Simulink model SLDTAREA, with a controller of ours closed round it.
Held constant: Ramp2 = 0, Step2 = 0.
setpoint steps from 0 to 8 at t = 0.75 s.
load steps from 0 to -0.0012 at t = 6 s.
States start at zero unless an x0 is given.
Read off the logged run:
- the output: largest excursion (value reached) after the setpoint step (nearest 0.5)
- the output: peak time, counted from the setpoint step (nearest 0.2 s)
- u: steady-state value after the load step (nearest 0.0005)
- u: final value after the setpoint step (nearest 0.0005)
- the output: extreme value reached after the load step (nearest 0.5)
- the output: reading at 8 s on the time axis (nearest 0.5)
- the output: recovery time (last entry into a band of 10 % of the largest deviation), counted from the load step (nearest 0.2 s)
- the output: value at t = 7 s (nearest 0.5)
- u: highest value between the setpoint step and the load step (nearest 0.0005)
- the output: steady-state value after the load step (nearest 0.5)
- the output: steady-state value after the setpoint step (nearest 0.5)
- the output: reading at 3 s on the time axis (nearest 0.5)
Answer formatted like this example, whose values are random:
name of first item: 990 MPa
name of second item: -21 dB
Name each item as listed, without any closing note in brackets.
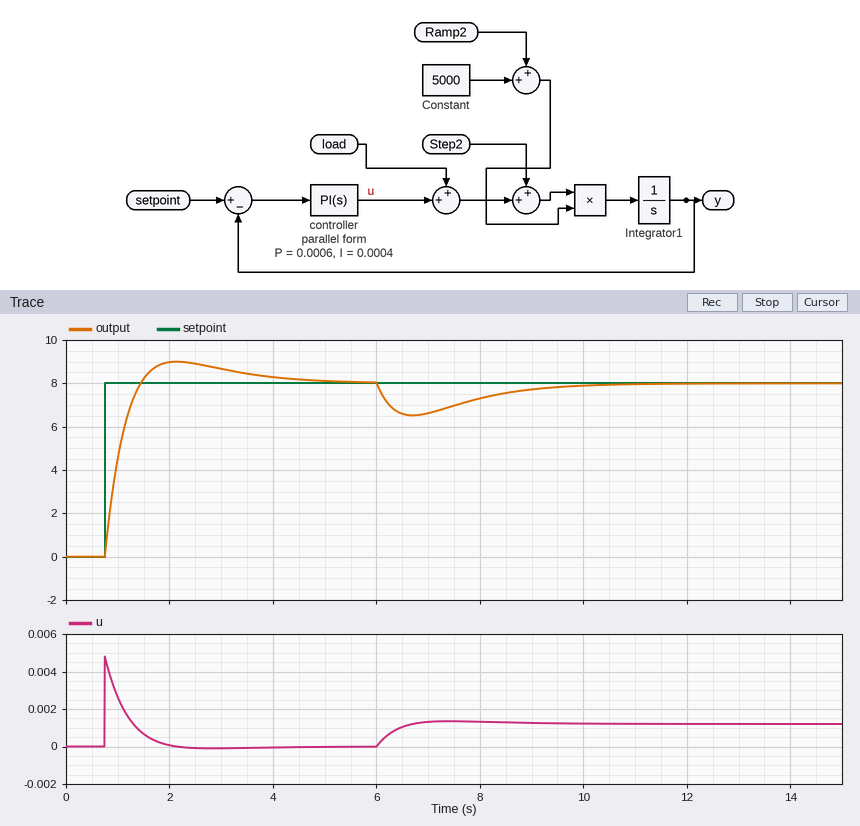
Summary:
the output: largest excursion (value reached) after the setpoint step: 9.0
the output: peak time, counted from the setpoint step: 1.4 s
u: steady-state value after the load step: 0.0010
u: final value after the setpoint step: 0.0000
the output: extreme value reached after the load step: 6.5
the output: reading at 8 s on the time axis: 7.5
the output: recovery time (last entry into a band of 10 % of the largest deviation), counted from the load step: 3.6 s
the output: value at t = 7 s: 6.5
u: highest value between the setpoint step and the load step: 0.0050
the output: steady-state value after the load step: 8.0
the output: steady-state value after the setpoint step: 8.0
the output: reading at 3 s on the time axis: 8.5
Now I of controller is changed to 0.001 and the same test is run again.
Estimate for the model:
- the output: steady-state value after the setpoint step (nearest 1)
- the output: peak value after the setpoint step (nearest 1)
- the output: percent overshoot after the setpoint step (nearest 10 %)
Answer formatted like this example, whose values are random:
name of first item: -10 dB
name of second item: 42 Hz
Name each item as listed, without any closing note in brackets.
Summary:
the output: steady-state value after the setpoint step: 8
the output: peak value after the setpoint step: 10
the output: percent overshoot after the setpoint step: 20 %
